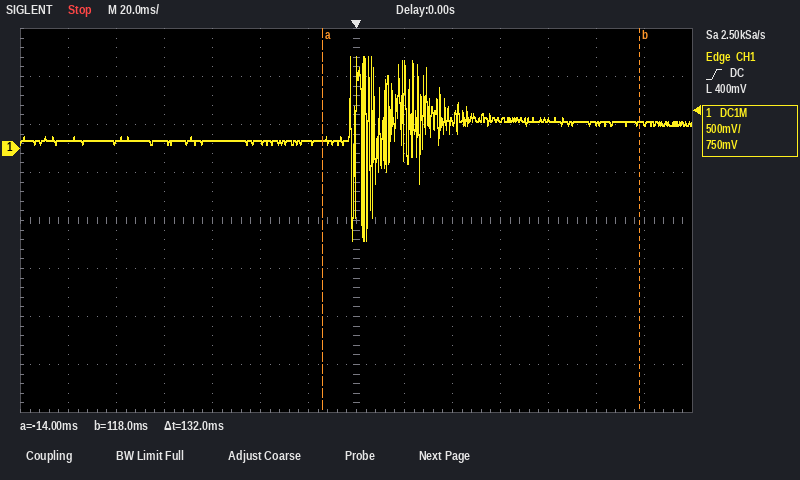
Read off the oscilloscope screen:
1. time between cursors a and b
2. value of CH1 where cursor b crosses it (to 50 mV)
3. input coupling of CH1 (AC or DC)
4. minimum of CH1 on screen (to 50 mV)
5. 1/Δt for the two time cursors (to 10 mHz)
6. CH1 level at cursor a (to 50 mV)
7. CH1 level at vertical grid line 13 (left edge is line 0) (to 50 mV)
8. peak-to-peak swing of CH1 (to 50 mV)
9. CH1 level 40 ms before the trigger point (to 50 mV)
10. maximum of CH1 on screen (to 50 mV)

132 ms
250 mV
DC
-950 mV
7.58 Hz
100 mV
250 mV
1.90 V
50 mV
950 mV
